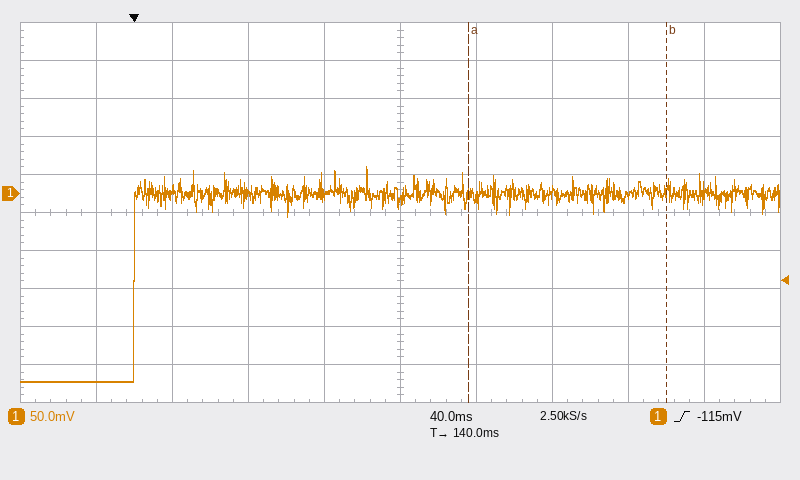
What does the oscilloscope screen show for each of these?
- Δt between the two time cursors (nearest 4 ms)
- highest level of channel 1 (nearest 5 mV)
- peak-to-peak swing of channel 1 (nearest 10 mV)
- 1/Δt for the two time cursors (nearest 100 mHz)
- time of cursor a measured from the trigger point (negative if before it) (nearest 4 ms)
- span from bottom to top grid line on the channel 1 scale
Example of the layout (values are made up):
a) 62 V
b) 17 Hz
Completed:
a) 104 ms
b) 35 mV
c) 280 mV
d) 9.6 Hz
e) +176 ms
f) 500 mV
